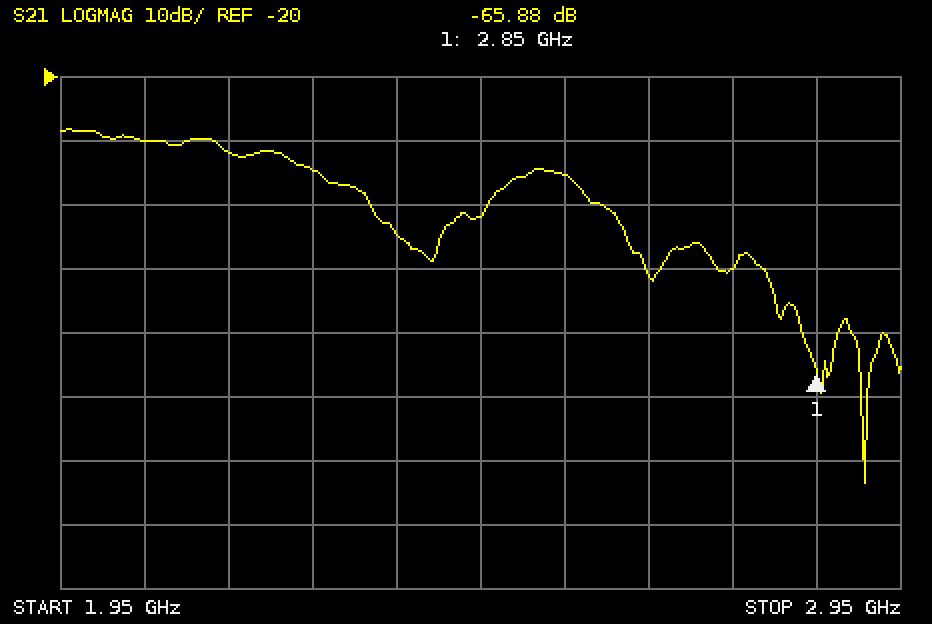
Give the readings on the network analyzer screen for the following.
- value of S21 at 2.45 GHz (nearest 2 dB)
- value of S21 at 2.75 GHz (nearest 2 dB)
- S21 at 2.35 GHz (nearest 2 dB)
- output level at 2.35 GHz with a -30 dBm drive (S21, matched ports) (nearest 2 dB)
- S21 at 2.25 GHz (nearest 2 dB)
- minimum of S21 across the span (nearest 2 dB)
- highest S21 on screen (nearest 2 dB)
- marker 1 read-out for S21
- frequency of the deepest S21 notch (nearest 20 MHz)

-42 dB
-50 dB
-44 dB
-74 dBm
-34 dB
-84 dB
-28 dB
-65.88 dB
2.90 GHz
